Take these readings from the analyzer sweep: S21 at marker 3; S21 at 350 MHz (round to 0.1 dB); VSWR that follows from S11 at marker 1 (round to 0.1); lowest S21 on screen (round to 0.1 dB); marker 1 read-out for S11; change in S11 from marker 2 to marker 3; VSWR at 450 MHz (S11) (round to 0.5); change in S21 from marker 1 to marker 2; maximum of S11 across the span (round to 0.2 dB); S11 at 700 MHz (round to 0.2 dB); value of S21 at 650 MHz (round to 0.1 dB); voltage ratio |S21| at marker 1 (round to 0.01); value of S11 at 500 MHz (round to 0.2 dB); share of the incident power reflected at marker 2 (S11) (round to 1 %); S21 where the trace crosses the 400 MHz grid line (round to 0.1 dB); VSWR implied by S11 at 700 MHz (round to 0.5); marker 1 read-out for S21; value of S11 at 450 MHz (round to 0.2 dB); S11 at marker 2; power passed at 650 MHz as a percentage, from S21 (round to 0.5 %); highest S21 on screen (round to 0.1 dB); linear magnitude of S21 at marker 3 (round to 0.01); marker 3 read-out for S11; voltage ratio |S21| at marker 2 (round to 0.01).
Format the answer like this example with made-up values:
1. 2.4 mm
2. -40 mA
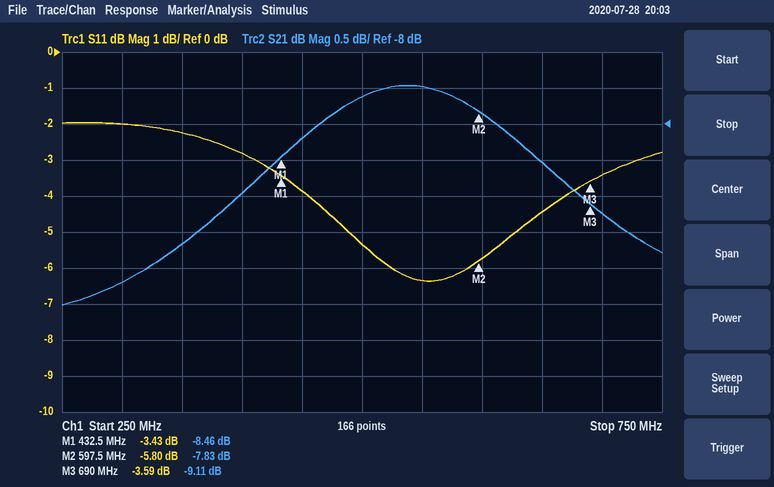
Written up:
1. -9.11 dB
2. -9.7 dB
3. 5.1
4. -10.5 dB
5. -3.43 dB
6. 2.21 dB
7. 4.5
8. 0.63 dB
9. -2.0 dB
10. -3.4 dB
11. -8.5 dB
12. 0.38
13. -5.4 dB
14. 26 %
15. -9.0 dB
16. 5.0
17. -8.46 dB
18. -3.8 dB
19. -5.80 dB
20. 14.0 %
21. -7.5 dB
22. 0.35
23. -3.59 dB
24. 0.41
